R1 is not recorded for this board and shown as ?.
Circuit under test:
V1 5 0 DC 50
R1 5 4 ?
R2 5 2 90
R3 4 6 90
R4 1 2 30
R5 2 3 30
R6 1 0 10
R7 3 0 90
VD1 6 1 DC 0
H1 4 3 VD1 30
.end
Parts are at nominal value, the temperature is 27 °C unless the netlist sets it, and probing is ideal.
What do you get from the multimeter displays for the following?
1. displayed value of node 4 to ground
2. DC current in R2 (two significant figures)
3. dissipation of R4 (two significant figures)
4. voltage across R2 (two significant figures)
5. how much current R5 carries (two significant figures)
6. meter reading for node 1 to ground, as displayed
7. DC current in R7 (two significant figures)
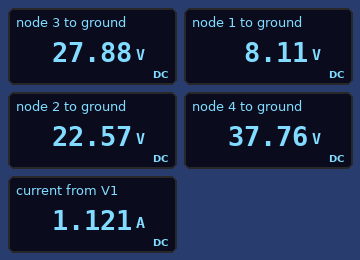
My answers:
37.76 V
300 mA
7.0 W
27 V
180 mA
8.11 V
310 mA
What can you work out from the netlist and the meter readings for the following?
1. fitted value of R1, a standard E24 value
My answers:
15 Ω
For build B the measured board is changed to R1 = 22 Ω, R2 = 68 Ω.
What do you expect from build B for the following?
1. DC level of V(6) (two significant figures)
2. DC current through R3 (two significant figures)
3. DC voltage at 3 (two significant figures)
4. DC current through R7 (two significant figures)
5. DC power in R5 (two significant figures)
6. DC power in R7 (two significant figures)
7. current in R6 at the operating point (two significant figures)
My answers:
8.0 V
300 mA
26 V
290 mA
300 mW
7.5 W
800 mA
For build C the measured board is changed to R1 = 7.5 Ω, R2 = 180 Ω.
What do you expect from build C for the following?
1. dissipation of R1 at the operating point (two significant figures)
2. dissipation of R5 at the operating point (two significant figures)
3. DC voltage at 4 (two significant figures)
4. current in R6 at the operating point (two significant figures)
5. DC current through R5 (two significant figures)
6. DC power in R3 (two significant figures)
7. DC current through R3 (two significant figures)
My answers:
7.8 W
2.7 W
42 V
830 mA
300 mA
13 W
380 mA
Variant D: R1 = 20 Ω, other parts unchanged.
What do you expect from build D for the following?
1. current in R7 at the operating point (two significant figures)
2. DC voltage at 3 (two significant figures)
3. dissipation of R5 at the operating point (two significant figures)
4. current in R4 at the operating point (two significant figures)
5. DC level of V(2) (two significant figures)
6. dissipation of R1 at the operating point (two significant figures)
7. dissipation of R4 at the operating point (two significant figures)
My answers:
290 mA
26 V
650 mW
460 mA
22 V
11 W
6.4 W
